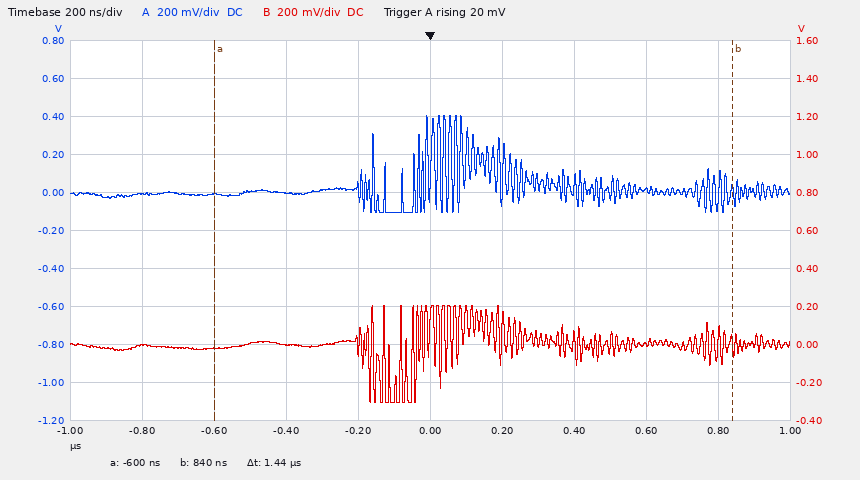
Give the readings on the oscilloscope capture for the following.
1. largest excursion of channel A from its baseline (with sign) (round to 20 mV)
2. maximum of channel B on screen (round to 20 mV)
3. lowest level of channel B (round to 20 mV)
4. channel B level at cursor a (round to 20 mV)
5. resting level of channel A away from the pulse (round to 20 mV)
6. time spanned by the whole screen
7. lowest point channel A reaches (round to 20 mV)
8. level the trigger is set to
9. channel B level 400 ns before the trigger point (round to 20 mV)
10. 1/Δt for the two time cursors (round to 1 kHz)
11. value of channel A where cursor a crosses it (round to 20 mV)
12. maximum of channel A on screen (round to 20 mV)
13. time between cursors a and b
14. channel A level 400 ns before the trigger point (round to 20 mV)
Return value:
+400 mV
200 mV
-300 mV
-20 mV
0 mV
2 µs
-100 mV
20 mV
0 mV
694 kHz
0 mV
400 mV
1.44 µs
0 mV
